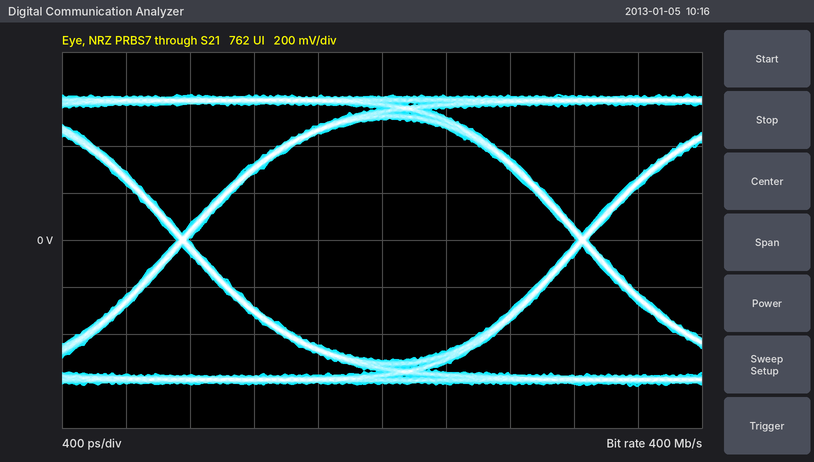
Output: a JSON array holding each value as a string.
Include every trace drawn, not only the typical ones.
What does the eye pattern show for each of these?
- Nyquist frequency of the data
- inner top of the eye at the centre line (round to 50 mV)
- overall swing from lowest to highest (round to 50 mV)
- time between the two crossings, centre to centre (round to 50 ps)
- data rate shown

["200 MHz", "500 mV", "1.25 V", "2.50 ns", "400 Mb/s"]
